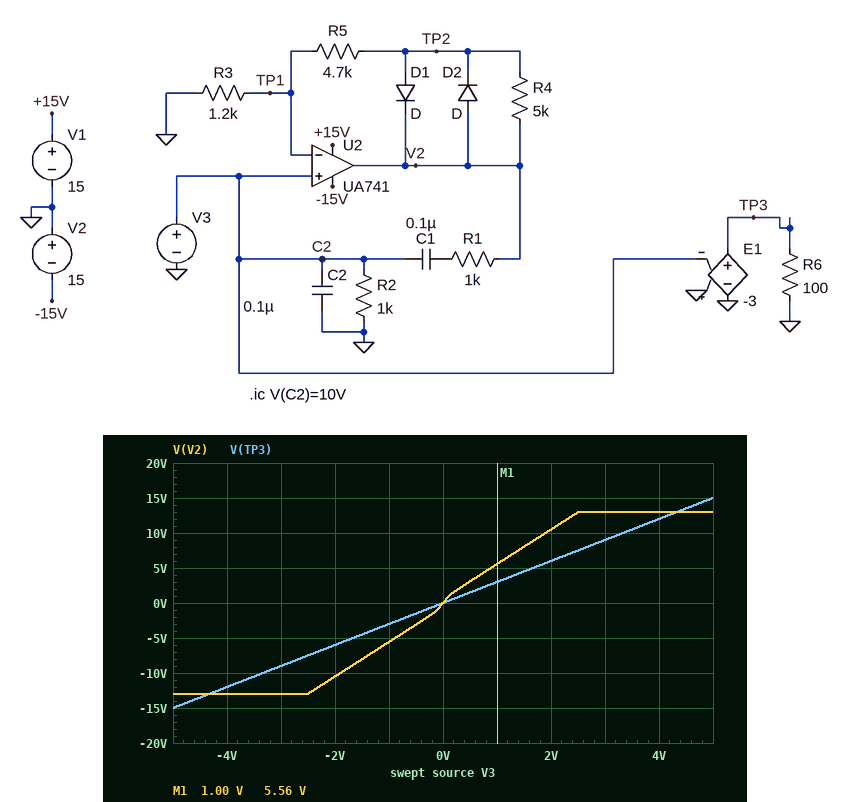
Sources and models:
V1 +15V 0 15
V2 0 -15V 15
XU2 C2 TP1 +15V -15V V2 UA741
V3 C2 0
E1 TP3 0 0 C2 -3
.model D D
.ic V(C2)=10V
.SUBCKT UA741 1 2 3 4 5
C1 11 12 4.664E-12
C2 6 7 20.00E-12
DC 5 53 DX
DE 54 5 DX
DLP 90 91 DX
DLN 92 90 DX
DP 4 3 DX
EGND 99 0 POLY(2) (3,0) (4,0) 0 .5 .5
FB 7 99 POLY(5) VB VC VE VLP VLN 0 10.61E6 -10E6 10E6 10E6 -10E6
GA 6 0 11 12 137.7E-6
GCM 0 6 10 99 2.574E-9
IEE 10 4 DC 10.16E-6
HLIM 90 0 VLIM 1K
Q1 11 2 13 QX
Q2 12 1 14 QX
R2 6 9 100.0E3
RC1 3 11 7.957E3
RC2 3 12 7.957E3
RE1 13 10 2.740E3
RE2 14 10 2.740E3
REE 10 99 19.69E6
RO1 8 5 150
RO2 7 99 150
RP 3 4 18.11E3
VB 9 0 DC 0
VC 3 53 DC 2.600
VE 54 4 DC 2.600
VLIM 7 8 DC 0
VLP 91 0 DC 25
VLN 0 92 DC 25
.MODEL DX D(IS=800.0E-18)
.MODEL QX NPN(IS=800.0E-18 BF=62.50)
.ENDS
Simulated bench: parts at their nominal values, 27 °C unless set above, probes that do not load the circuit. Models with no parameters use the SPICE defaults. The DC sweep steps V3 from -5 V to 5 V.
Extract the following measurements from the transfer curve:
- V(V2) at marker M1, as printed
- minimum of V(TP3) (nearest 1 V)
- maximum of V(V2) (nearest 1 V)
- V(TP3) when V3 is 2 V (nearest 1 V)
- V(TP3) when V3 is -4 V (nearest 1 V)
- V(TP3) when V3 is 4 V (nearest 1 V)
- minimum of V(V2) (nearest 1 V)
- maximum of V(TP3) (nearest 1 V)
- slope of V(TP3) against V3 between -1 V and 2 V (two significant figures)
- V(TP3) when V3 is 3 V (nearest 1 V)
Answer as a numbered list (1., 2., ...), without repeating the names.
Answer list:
1. 5.56 V
2. -15 V
3. 13 V
4. 6 V
5. -12 V
6. 12 V
7. -13 V
8. 15 V
9. 3.0 V/V
10. 9 V
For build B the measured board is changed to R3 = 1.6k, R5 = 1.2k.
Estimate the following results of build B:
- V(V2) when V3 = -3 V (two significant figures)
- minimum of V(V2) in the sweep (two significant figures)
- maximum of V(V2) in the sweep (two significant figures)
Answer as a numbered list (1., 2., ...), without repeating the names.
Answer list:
1. -5.9 V
2. -9.4 V
3. 9.4 V
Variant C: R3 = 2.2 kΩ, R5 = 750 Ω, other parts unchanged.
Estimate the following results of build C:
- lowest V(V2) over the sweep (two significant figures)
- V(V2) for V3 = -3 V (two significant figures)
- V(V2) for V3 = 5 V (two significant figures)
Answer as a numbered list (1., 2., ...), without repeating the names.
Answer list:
1. -7.4 V
2. -4.7 V
3. 7.4 V
